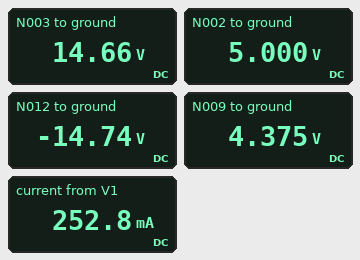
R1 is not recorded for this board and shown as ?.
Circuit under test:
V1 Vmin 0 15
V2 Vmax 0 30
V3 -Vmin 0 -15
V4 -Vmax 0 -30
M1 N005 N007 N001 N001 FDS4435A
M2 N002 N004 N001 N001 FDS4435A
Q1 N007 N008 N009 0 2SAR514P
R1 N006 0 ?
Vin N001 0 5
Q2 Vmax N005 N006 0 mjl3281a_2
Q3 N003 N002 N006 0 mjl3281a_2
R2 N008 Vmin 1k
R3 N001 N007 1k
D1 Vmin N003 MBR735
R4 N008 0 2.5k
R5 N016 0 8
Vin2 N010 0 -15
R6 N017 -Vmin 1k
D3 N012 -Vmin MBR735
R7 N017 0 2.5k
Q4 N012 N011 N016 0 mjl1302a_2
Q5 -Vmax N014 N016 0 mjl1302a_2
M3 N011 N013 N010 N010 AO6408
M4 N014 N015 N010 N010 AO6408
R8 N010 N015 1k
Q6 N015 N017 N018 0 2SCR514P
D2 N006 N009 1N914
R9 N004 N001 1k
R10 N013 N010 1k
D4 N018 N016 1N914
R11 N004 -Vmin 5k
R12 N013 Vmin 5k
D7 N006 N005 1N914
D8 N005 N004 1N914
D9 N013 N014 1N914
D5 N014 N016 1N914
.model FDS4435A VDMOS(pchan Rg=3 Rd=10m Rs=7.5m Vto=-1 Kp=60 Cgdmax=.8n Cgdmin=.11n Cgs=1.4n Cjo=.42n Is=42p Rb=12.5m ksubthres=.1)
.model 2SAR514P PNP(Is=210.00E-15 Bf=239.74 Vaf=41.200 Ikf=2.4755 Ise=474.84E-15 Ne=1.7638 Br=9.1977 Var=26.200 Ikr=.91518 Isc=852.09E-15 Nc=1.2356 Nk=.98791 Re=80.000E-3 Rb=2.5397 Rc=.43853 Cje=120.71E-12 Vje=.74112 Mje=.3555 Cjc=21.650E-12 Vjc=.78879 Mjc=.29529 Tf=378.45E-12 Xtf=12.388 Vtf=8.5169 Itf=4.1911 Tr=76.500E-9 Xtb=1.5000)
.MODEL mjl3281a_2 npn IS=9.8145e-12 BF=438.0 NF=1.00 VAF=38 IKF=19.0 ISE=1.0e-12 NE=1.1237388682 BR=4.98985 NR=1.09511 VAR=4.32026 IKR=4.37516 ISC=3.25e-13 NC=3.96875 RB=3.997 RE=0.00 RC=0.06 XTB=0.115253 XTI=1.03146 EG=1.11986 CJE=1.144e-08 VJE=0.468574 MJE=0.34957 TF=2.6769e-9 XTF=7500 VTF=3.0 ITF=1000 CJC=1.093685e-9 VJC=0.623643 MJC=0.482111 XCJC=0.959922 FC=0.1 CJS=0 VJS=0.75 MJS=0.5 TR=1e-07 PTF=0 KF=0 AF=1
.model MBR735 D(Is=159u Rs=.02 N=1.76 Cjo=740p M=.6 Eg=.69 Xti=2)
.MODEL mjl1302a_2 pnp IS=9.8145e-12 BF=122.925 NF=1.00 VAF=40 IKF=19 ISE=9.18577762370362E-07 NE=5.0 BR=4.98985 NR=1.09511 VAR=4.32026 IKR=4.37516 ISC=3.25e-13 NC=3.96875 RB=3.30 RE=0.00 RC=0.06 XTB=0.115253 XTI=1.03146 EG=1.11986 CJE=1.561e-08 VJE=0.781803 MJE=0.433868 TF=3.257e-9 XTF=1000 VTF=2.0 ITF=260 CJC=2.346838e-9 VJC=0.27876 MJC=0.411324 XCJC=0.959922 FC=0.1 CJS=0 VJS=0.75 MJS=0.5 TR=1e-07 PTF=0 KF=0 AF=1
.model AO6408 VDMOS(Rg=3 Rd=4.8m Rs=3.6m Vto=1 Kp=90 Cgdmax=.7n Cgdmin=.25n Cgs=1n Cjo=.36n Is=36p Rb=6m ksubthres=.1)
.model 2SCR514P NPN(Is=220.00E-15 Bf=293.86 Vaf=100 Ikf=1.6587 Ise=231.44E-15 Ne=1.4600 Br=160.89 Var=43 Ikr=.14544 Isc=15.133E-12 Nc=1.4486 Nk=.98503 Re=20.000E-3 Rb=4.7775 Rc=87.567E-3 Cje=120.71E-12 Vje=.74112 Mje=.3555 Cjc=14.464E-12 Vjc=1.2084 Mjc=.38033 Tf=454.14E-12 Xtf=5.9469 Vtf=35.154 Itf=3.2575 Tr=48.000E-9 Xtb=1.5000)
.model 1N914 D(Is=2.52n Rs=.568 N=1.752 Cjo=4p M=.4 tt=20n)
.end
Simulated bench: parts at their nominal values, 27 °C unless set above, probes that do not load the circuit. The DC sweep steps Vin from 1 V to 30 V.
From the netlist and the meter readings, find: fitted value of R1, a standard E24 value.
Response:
18 Ω
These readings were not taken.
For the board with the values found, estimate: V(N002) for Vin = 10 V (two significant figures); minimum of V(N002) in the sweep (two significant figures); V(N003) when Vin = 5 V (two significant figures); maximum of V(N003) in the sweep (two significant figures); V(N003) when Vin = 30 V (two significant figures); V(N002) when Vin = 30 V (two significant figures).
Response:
10 V
1.0 V
15 V
29 V
29 V
30 V
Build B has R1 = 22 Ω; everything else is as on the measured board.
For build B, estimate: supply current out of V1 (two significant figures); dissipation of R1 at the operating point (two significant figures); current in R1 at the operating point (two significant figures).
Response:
210 mA
870 mW
200 mA
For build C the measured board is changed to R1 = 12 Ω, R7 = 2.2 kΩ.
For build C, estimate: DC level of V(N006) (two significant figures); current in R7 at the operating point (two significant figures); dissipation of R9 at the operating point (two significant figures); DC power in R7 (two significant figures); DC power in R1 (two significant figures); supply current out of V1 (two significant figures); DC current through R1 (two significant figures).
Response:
4.4 V
5.9 mA
3.5 mW
76 mW
1.6 W
370 mA
360 mA
